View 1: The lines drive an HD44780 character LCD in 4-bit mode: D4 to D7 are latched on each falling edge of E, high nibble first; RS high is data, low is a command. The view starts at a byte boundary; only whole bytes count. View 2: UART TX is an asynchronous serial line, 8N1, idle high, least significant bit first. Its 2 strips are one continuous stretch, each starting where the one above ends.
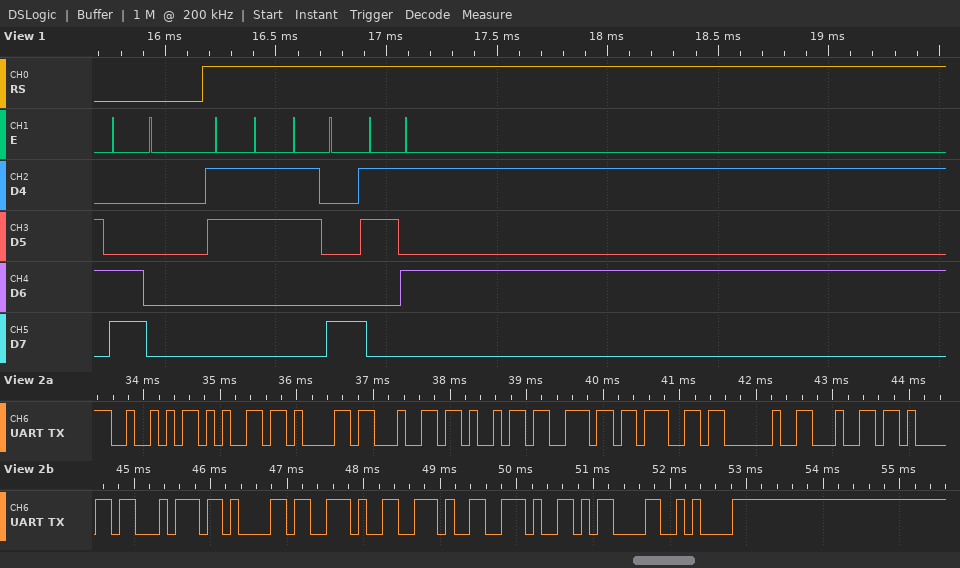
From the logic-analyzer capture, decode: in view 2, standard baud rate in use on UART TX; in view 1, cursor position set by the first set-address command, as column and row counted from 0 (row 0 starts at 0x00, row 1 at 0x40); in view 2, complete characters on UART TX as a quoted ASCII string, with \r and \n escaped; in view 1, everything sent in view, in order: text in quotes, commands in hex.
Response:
9600 baud
column 0, row 1
"Reading data...\r\n"
0xC0 "385"
